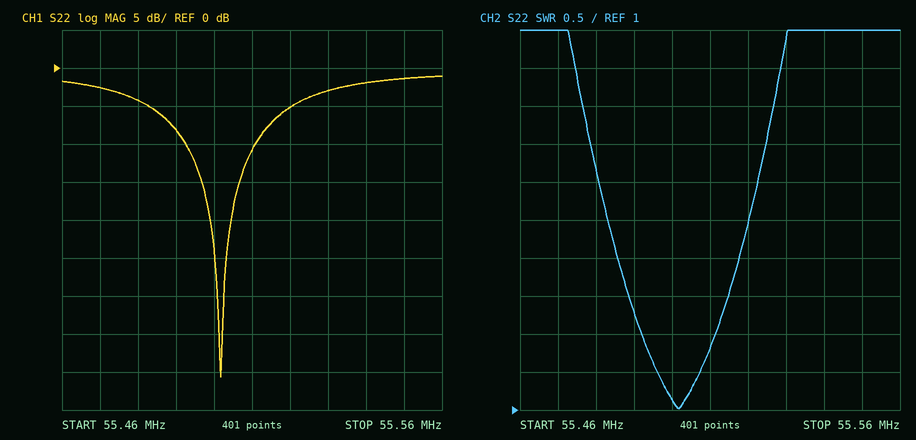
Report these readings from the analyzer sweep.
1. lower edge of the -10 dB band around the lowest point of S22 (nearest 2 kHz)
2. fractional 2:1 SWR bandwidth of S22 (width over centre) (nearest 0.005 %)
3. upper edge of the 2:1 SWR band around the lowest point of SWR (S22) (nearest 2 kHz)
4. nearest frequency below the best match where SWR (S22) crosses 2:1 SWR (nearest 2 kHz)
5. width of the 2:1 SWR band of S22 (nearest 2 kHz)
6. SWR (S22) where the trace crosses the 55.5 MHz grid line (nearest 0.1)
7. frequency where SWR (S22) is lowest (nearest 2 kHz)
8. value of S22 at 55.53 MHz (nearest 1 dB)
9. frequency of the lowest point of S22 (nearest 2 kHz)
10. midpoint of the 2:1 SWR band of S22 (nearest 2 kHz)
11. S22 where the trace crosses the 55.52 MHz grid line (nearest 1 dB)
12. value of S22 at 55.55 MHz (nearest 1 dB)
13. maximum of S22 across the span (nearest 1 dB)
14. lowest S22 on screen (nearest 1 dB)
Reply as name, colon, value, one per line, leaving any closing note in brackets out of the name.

lower edge of the -10 dB band around the lowest point of S22: 55.492 MHz
fractional 2:1 SWR bandwidth of S22 (width over centre): 0.035 %
upper edge of the 2:1 SWR band around the lowest point of SWR (S22): 55.512 MHz
nearest frequency below the best match where SWR (S22) crosses 2:1 SWR: 55.492 MHz
width of the 2:1 SWR band of S22: 20 kHz
SWR (S22) where the trace crosses the 55.5 MHz grid line: 1.1
frequency where SWR (S22) is lowest: 55.502 MHz
value of S22 at 55.53 MHz: -3 dB
frequency of the lowest point of S22: 55.502 MHz
midpoint of the 2:1 SWR band of S22: 55.502 MHz
S22 where the trace crosses the 55.52 MHz grid line: -5 dB
value of S22 at 55.55 MHz: -1 dB
maximum of S22 across the span: -1 dB
lowest S22 on screen: -41 dB
